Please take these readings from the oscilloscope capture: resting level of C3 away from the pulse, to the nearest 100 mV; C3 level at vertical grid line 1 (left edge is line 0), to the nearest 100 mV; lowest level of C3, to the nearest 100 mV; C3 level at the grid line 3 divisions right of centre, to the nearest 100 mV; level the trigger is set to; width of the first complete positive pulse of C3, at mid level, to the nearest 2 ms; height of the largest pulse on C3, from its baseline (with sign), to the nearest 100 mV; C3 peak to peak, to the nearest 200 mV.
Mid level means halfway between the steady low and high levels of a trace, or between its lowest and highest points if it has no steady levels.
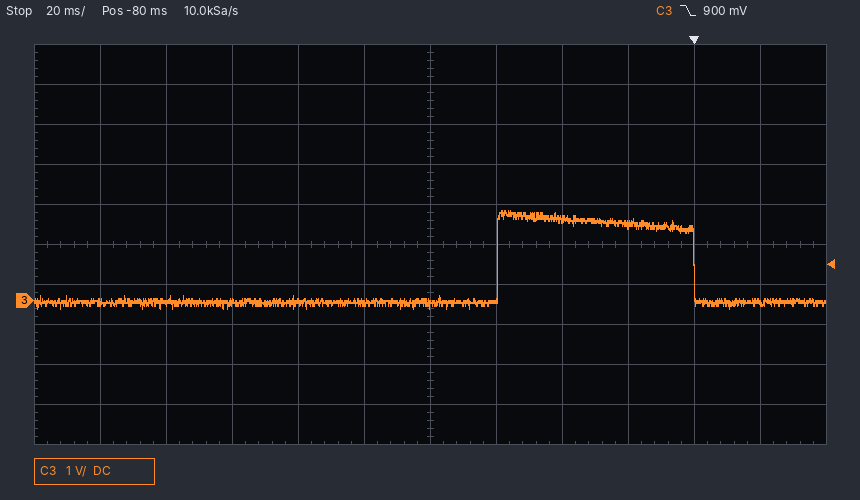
0.0 V
0.0 V
-200 mV
1.9 V
900 mV
60 ms
+2.3 V
2.4 V
